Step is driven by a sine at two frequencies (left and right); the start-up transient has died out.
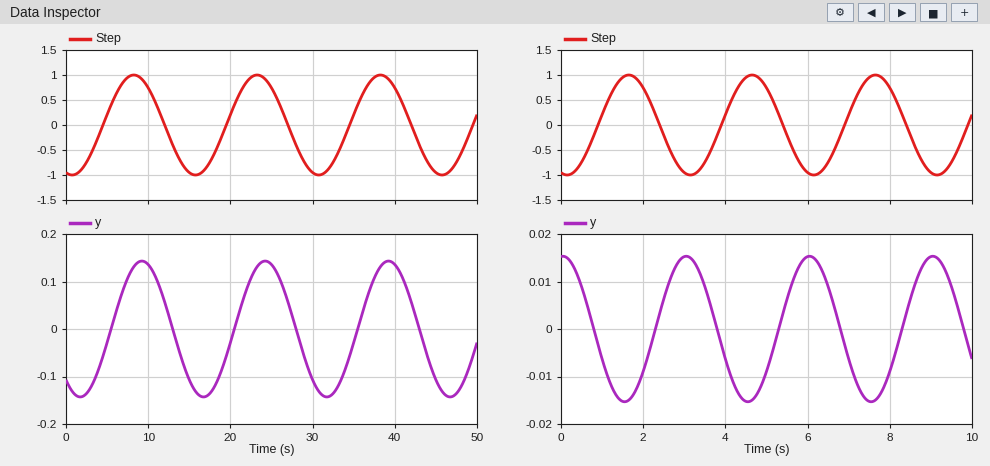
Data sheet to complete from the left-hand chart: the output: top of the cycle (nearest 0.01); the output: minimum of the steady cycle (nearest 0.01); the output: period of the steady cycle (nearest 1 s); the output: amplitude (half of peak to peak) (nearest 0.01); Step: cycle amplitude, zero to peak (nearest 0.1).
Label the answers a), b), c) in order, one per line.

a) 0.14
b) -0.14
c) 15 s
d) 0.14
e) 1.0
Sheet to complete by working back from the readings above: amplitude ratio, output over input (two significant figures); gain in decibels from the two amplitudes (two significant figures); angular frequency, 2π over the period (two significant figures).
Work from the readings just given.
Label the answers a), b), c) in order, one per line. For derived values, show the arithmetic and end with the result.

a) 0.14 / 1 = 0.14
b) 20 log10(0.14 / 1) = -17 dB
c) 2π / 15 = 0.42 rad/s
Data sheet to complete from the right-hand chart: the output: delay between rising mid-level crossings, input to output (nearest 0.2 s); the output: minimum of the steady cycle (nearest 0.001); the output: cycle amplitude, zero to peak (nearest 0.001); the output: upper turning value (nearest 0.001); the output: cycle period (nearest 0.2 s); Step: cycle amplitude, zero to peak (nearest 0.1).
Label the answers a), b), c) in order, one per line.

a) 1.4 s
b) -0.015
c) 0.015
d) 0.015
e) 3.0 s
f) 1.0
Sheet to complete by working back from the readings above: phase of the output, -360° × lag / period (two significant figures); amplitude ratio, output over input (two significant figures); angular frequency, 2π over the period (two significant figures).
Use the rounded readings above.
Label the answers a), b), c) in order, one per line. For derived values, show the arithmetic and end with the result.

a) -360 × 1.4 / 3 = -170°
b) 0.015 / 1 = 0.015
c) 2π / 3 = 2.1 rad/s
